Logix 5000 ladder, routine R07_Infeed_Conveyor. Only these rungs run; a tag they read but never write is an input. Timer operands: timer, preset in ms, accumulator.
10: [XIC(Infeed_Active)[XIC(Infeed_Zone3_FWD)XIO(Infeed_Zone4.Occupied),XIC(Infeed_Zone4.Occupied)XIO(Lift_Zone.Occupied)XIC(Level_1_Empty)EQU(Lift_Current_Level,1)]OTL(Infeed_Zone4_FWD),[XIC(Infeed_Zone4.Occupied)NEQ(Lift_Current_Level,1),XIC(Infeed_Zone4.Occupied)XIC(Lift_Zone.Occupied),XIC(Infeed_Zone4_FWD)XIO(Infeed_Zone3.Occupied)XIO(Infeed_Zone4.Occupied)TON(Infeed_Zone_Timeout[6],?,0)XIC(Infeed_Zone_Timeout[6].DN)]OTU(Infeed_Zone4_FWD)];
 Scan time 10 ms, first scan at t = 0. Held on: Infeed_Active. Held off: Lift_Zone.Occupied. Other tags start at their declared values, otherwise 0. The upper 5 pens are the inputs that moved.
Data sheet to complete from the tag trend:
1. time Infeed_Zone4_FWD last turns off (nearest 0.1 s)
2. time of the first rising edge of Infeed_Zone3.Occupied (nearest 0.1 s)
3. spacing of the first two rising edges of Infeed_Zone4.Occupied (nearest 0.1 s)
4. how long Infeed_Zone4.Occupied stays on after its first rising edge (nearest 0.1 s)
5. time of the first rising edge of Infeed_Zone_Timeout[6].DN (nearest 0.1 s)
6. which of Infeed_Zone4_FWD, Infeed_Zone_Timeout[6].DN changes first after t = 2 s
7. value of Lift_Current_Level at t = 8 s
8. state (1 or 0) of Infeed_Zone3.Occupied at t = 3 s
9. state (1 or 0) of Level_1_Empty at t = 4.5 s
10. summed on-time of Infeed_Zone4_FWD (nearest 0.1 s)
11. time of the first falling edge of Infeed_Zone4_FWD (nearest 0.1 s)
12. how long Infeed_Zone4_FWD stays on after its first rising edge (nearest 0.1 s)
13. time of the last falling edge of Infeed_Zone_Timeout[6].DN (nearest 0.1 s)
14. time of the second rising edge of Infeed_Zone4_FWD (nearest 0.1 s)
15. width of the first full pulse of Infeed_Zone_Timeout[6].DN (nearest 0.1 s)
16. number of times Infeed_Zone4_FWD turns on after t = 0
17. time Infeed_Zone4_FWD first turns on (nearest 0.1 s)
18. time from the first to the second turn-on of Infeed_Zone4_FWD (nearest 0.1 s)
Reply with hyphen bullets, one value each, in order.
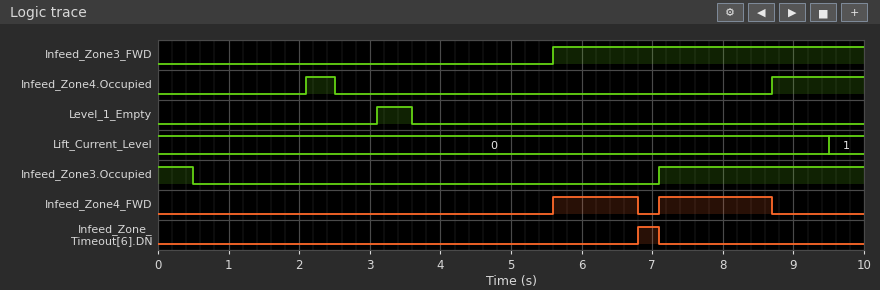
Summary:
- 8.7 s
- 7.1 s
- 6.6 s
- 0.4 s
- 6.8 s
- Infeed_Zone4_FWD
- 0
- 0
- 0
- 2.8 s
- 6.8 s
- 1.2 s
- 7.1 s
- 7.1 s
- 0.3 s
- 2
- 5.6 s
- 1.5 s
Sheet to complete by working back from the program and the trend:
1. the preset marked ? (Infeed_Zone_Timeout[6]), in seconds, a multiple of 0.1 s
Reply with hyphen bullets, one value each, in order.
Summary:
- 1.2 s
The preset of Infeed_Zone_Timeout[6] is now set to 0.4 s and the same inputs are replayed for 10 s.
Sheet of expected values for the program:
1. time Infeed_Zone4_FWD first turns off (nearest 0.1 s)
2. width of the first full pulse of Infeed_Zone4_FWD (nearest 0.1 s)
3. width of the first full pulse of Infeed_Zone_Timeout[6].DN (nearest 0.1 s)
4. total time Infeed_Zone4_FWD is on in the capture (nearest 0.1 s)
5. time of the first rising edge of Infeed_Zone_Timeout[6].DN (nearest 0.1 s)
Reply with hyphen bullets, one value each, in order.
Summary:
- 6.0 s
- 0.4 s
- 1.1 s
- 2.0 s
- 6.0 s
